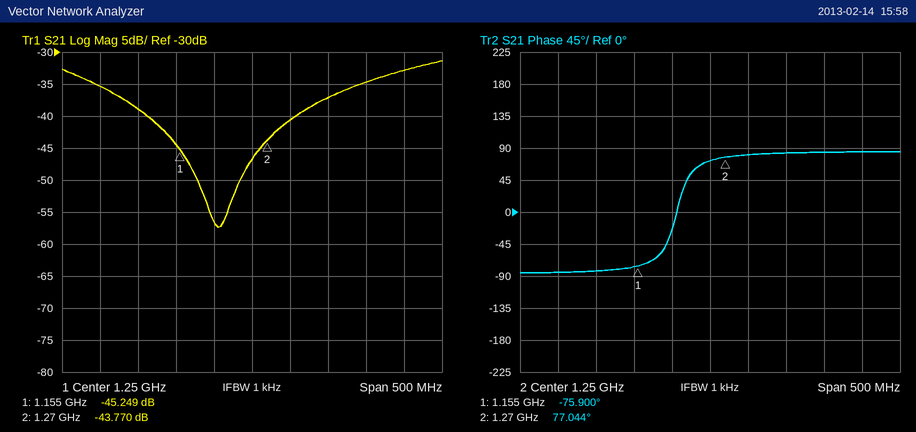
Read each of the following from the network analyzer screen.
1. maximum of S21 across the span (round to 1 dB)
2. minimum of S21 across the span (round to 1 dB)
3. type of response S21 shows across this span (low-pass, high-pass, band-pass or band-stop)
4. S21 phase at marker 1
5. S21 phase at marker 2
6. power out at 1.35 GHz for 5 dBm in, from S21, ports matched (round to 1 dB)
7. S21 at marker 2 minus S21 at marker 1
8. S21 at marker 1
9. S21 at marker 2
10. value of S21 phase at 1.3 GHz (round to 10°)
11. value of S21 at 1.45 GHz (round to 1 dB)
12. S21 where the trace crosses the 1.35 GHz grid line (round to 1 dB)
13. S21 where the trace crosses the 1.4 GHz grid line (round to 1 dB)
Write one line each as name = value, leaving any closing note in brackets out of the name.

maximum of S21 across the span = -31 dB
minimum of S21 across the span = -57 dB
type of response S21 shows across this span = band-stop
S21 phase at marker 1 = -75.900°
S21 phase at marker 2 = 77.044°
power out at 1.35 GHz for 5 dBm in, from S21, ports matched = -32 dBm
S21 at marker 2 minus S21 at marker 1 = 1.479 dB
S21 at marker 1 = -45.249 dB
S21 at marker 2 = -43.770 dB
value of S21 phase at 1.3 GHz = 80°
value of S21 at 1.45 GHz = -33 dB
S21 where the trace crosses the 1.35 GHz grid line = -37 dB
S21 where the trace crosses the 1.4 GHz grid line = -35 dB
